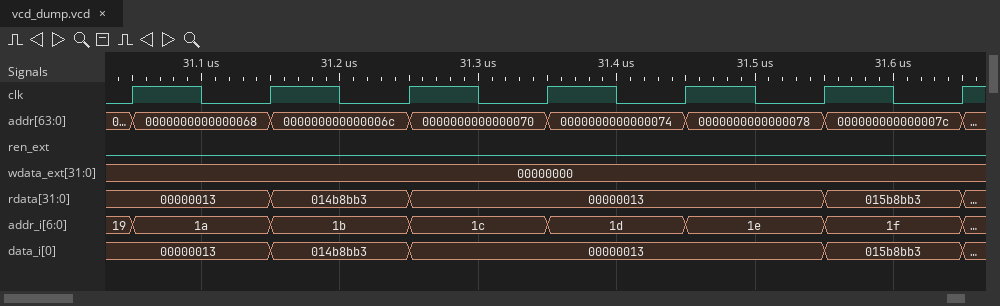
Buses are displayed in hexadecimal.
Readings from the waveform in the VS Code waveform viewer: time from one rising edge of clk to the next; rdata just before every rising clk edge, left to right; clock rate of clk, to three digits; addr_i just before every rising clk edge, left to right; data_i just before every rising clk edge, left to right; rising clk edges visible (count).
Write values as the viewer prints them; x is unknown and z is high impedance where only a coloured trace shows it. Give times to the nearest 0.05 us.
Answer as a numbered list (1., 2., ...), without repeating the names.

1. 0.1 us
2. 00000013, 00000013, 014b8bb3, 00000013, 00000013, 00000013, 015b8bb3
3. 10.0 MHz
4. 19, 1a, 1b, 1c, 1d, 1e, 1f
5. 00000013, 00000013, 014b8bb3, 00000013, 00000013, 00000013, 015b8bb3
6. 7
